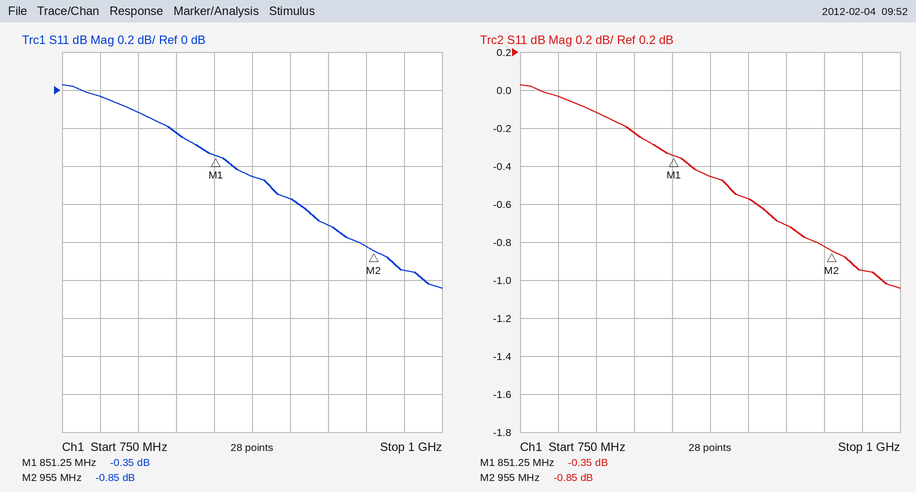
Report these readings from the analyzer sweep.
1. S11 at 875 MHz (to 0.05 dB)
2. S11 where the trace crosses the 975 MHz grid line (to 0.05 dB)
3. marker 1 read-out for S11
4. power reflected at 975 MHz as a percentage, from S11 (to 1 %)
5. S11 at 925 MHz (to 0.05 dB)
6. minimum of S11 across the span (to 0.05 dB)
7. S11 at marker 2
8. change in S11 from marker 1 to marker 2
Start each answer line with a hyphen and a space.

- -0.45 dB
- -0.95 dB
- -0.35 dB
- 80 %
- -0.70 dB
- -1.05 dB
- -0.85 dB
- -0.50 dB
